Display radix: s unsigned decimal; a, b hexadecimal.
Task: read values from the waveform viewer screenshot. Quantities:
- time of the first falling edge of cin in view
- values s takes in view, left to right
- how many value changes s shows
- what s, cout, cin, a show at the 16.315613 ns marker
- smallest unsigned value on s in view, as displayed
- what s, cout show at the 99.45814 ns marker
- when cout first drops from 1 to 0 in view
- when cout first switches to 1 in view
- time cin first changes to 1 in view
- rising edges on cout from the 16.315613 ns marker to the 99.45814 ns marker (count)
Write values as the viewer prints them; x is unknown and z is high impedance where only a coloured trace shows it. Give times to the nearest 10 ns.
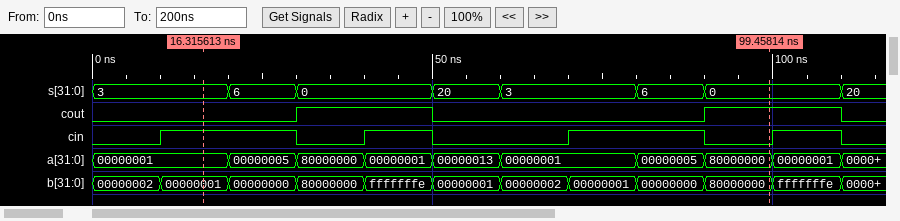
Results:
30 ns
3, 6, 0, 20, 3, 6, 0, 20
7
s=3, cout=0, cin=1, a=00000001
0
s=0, cout=1
50 ns
30 ns
10 ns
2
